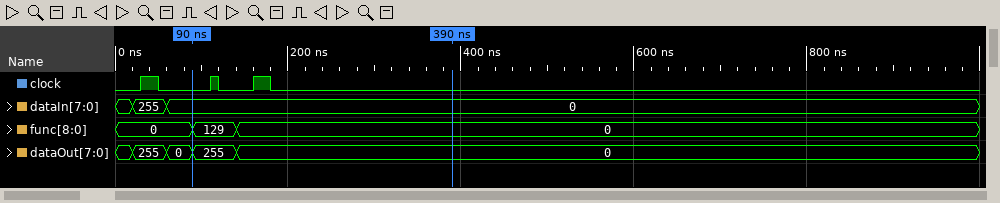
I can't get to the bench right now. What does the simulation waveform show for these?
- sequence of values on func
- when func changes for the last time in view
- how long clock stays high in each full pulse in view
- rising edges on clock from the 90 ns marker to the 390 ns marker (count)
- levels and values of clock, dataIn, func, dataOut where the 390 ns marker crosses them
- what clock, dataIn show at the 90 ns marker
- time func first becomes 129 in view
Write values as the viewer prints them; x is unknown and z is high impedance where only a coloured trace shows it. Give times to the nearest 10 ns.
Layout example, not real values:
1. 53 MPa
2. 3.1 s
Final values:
1. 0, 129, 0
2. 140 ns
3. 20 ns, 10 ns, 20 ns
4. 2
5. clock=0, dataIn=0, func=0, dataOut=0
6. clock=0, dataIn=0
7. 90 ns
